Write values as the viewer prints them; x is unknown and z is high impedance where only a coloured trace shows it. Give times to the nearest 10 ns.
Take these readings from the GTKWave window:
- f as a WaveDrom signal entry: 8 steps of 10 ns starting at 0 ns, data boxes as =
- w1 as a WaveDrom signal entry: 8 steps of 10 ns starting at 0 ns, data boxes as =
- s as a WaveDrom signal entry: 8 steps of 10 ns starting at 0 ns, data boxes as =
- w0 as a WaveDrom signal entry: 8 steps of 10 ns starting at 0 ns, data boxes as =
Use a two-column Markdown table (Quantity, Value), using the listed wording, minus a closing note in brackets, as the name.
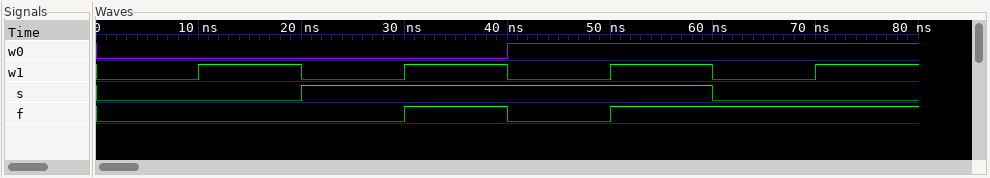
| Quantity | Value |
|---|---|
| f as a WaveDrom signal entry: 8 steps of 10 ns starting at 0 ns, data boxes as = | {name: 'f', wave: '0..101..'} |
| w1 as a WaveDrom signal entry: 8 steps of 10 ns starting at 0 ns, data boxes as = | {name: 'w1', wave: '01010101'} |
| s as a WaveDrom signal entry: 8 steps of 10 ns starting at 0 ns, data boxes as = | {name: 's', wave: '0.1...0.'} |
| w0 as a WaveDrom signal entry: 8 steps of 10 ns starting at 0 ns, data boxes as = | {name: 'w0', wave: '0...1...'} |
